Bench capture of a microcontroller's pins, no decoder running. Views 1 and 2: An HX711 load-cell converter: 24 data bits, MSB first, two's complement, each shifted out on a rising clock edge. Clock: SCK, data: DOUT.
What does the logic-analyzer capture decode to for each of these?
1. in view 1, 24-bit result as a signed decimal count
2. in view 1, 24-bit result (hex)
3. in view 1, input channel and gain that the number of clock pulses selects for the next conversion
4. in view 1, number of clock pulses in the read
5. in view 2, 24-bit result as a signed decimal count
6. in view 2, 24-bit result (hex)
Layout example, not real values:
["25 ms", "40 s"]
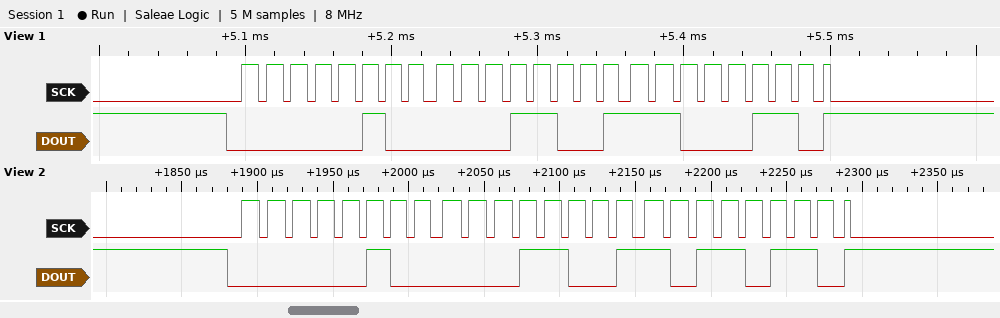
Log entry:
["268742", "0x0419C6", "channel A, gain 128", "25", "268726", "0x0419B6"]
